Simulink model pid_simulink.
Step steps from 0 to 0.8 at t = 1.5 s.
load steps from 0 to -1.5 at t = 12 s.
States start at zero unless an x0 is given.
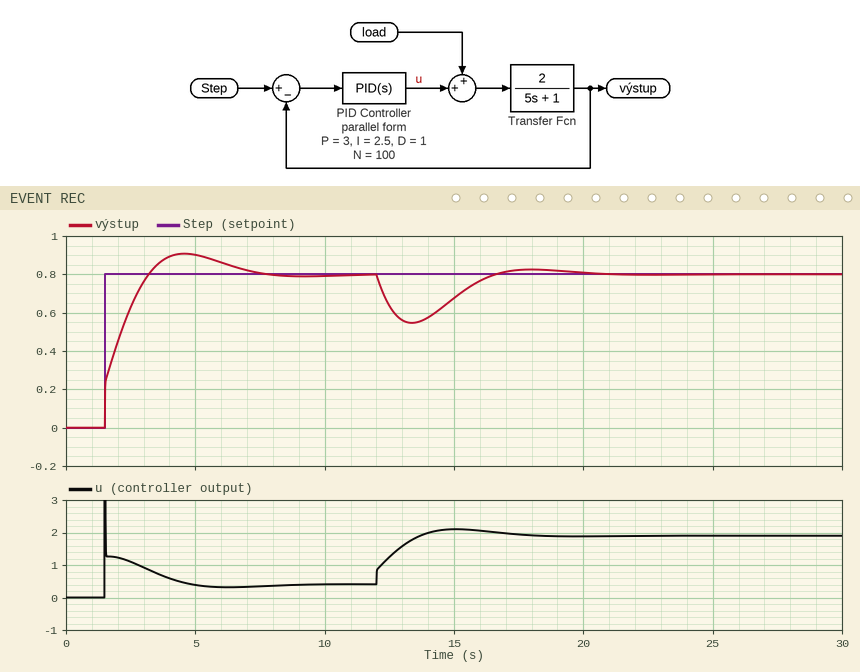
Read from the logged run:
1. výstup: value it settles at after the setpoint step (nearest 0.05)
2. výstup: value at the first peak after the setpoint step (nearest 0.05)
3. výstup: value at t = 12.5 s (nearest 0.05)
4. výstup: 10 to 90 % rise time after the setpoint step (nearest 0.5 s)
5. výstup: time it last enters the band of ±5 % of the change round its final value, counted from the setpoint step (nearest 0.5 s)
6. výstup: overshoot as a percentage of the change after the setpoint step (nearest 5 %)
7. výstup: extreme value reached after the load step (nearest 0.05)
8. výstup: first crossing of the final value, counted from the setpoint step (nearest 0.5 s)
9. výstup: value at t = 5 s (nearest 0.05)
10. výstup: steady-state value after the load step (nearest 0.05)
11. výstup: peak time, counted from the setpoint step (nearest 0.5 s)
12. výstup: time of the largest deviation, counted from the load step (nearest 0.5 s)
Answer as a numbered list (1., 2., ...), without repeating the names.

1. 0.80
2. 0.90
3. 0.65
4. 1.5 s
5. 5.0 s
6. 15 %
7. 0.55
8. 1.5 s
9. 0.90
10. 0.80
11. 3.0 s
12. 1.5 s
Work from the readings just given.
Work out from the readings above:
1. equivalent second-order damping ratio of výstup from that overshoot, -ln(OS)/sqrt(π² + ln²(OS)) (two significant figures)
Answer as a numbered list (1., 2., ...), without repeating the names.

1. 0.52
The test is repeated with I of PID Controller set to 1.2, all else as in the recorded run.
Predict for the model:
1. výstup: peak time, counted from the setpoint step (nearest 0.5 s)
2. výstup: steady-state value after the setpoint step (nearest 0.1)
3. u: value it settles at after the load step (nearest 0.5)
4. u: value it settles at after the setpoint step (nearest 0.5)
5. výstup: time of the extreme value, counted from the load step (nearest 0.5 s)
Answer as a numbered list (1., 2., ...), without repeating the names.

1. 4.5 s
2. 0.8
3. 2.0
4. 0.5
5. 2.0 s
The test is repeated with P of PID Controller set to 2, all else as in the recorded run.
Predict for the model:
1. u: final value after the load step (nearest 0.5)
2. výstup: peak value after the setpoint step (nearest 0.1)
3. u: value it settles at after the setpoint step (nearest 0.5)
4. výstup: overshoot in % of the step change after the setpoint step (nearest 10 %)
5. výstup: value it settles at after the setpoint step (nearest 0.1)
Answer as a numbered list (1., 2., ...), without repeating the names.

1. 2.0
2. 1.0
3. 0.5
4. 20 %
5. 0.8
